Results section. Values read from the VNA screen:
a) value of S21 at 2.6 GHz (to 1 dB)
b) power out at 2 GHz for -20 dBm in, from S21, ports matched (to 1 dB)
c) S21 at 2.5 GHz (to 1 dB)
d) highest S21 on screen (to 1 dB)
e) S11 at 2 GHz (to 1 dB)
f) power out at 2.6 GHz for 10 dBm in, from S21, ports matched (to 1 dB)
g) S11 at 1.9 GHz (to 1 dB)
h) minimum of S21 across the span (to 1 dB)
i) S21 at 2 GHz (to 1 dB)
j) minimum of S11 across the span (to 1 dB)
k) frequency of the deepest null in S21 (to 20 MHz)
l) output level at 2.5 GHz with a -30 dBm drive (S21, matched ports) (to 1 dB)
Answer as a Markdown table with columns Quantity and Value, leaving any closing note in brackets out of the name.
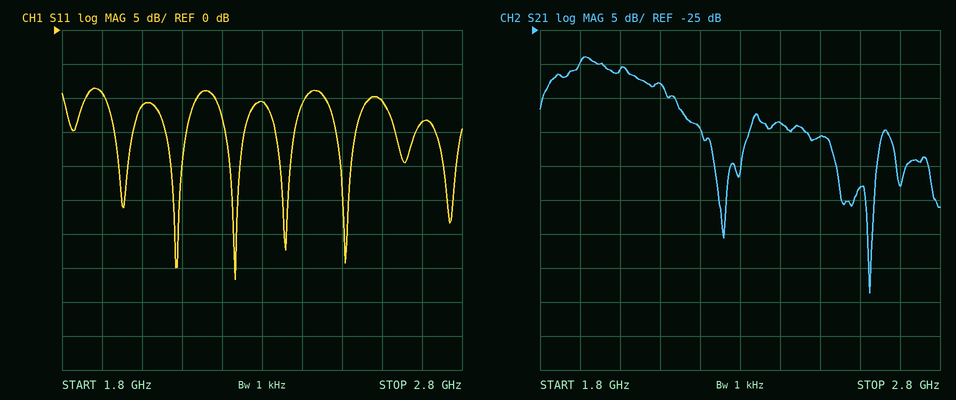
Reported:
| Quantity | Value |
|---|---|
| value of S21 at 2.6 GHz | -48 dB |
| power out at 2 GHz for -20 dBm in, from S21, ports matched | -51 dBm |
| S21 at 2.5 GHz | -41 dB |
| highest S21 on screen | -29 dB |
| S11 at 2 GHz | -11 dB |
| power out at 2.6 GHz for 10 dBm in, from S21, ports matched | -38 dBm |
| S11 at 1.9 GHz | -9 dB |
| minimum of S21 across the span | -64 dB |
| S21 at 2 GHz | -31 dB |
| minimum of S11 across the span | -37 dB |
| frequency of the deepest null in S21 | 2.62 GHz |
| output level at 2.5 GHz with a -30 dBm drive (S21, matched ports) | -71 dBm |
